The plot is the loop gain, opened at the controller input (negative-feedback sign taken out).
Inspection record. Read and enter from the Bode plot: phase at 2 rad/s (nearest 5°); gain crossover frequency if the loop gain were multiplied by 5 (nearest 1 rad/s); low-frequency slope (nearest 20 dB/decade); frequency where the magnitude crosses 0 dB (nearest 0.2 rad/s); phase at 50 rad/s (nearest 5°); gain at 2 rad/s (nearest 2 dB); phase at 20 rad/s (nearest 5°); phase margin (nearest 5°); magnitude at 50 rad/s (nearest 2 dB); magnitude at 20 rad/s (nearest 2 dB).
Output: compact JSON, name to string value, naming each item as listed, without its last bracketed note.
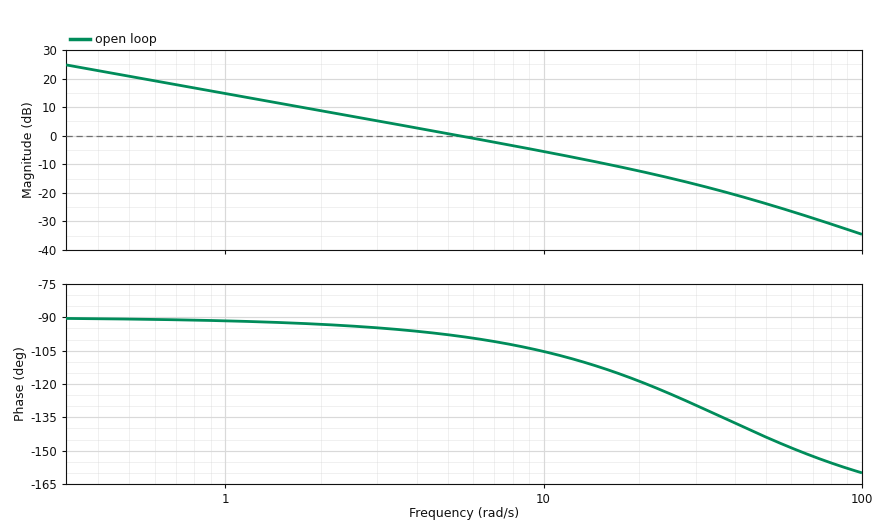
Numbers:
{"phase at 2 rad/s": "-95°", "gain crossover frequency if the loop gain were multiplied by 5": "23 rad/s", "low-frequency slope": "-20 dB/decade", "frequency where the magnitude crosses 0 dB": "5.4 rad/s", "phase at 50 rad/s": "-145°", "gain at 2 rad/s": "8 dB", "phase at 20 rad/s": "-120°", "phase margin": "80°", "magnitude at 50 rad/s": "-24 dB", "magnitude at 20 rad/s": "-12 dB"}
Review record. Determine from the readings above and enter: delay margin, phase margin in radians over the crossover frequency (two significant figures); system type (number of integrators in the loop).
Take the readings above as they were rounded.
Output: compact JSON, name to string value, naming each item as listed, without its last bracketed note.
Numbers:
{"delay margin, phase margin in radians over the crossover frequency": "0.26 s", "system type": "1"}
